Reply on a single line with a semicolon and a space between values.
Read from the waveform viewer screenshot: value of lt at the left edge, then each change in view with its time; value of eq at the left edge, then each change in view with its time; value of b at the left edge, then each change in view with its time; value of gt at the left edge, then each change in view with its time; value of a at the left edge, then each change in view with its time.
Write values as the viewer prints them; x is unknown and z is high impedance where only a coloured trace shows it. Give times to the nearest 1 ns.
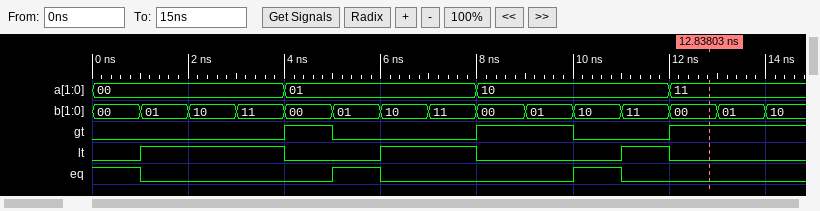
0, 1 at 1 ns, 0 at 4 ns, 1 at 6 ns, 0 at 8 ns, 1 at 11 ns, 0 at 12 ns; 1, 0 at 1 ns, 1 at 5 ns, 0 at 6 ns, 1 at 10 ns, 0 at 11 ns; 00, 01 at 1 ns, 10 at 2 ns, 11 at 3 ns, 00 at 4 ns, 01 at 5 ns, 10 at 6 ns, 11 at 7 ns, 00 at 8 ns, 01 at 9 ns, 10 at 10 ns, 11 at 11 ns, 00 at 12 ns, 01 at 13 ns, 10 at 14 ns; 0, 1 at 4 ns, 0 at 5 ns, 1 at 8 ns, 0 at 10 ns, 1 at 12 ns; 00, 01 at 4 ns, 10 at 8 ns, 11 at 12 ns
